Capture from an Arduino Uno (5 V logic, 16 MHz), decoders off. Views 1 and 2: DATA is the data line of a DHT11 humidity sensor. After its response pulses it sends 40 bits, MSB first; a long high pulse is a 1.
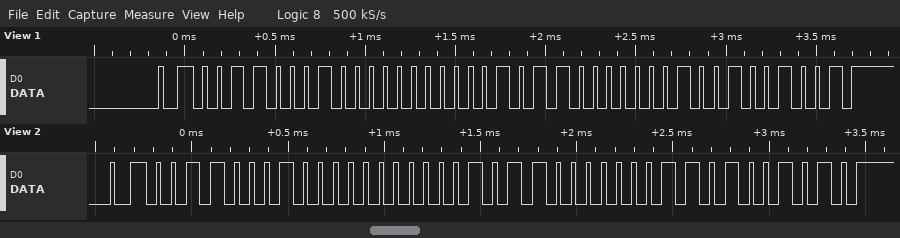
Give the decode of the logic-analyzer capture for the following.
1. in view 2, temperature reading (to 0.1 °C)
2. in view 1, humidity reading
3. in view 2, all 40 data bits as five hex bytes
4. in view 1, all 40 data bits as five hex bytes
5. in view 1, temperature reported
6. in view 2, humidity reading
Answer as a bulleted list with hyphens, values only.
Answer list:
- 22.3 °C
- 49 %
- 31 00 16 03 4A
- 31 00 16 02 49
- 22.2 °C
- 49 %
